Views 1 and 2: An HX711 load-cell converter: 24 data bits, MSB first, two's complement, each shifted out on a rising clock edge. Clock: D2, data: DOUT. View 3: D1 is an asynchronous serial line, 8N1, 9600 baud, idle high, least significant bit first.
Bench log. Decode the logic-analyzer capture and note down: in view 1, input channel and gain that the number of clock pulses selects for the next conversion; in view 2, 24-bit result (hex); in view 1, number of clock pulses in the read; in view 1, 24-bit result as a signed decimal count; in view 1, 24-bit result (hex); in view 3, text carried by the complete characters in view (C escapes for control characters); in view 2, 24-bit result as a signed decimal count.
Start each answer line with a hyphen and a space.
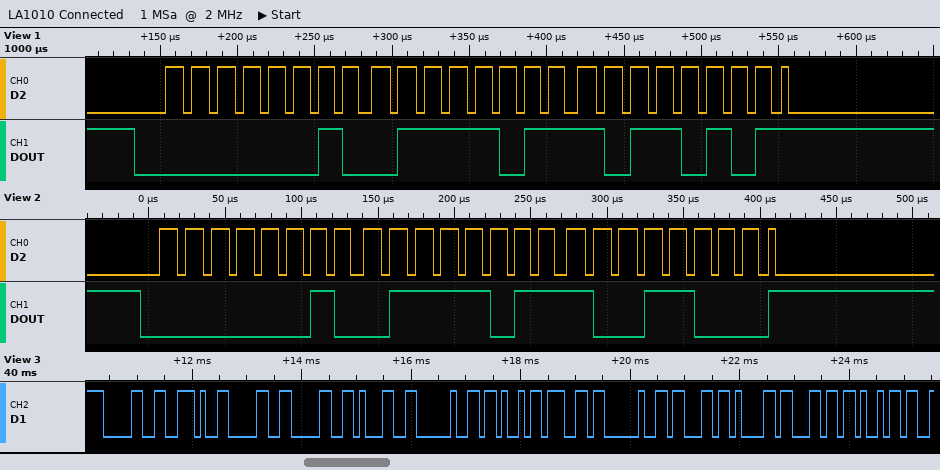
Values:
- channel A, gain 128
- 0x027B98
- 25
- 162741
- 0x027BB5
- "0.001 Kg cali"
- 162712
